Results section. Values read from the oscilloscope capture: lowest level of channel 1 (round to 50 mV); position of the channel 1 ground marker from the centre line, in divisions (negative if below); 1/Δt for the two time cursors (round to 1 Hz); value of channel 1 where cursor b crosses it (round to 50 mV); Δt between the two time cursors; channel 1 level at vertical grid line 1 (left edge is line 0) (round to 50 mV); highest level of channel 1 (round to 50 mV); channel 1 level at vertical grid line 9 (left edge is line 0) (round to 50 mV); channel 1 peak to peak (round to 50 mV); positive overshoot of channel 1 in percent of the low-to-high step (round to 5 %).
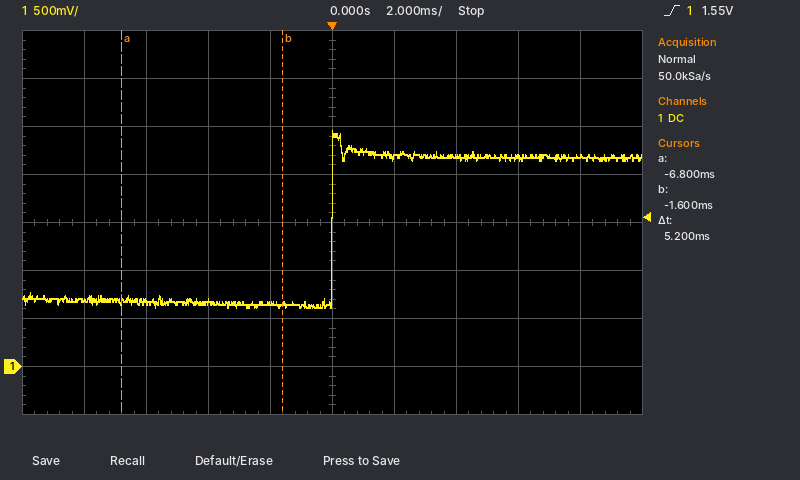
600 mV
-3.0 div
192 Hz
650 mV
5.2 ms
700 mV
2.45 V
2.20 V
1.85 V
20 %
